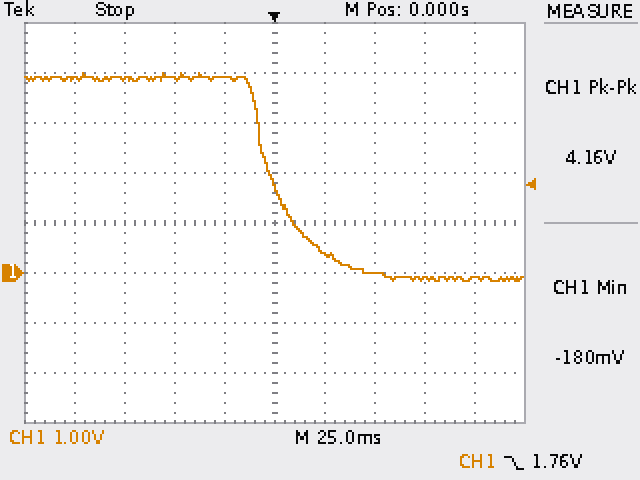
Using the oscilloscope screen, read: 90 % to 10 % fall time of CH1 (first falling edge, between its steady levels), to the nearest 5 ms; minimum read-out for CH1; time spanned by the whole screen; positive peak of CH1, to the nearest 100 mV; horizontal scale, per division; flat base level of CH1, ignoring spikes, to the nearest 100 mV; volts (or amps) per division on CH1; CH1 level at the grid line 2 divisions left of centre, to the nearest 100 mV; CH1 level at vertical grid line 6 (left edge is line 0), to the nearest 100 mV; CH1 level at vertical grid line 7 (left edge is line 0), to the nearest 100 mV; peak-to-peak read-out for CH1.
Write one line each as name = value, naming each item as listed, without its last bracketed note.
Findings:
90 % to 10 % fall time of CH1 (first falling edge, between its steady levels), to the nearest 5 ms = 40 ms
minimum read-out for CH1 = -180 mV
time spanned by the whole screen = 250 ms
positive peak of CH1, to the nearest 100 mV = 4.0 V
horizontal scale, per division = 25 ms
flat base level of CH1, ignoring spikes, to the nearest 100 mV = -100 mV
volts (or amps) per division on CH1 = 1 V
CH1 level at the grid line 2 divisions left of centre, to the nearest 100 mV = 3.9 V
CH1 level at vertical grid line 6 (left edge is line 0), to the nearest 100 mV = 400 mV
CH1 level at vertical grid line 7 (left edge is line 0), to the nearest 100 mV = 0.0 V
peak-to-peak read-out for CH1 = 4.16 V
